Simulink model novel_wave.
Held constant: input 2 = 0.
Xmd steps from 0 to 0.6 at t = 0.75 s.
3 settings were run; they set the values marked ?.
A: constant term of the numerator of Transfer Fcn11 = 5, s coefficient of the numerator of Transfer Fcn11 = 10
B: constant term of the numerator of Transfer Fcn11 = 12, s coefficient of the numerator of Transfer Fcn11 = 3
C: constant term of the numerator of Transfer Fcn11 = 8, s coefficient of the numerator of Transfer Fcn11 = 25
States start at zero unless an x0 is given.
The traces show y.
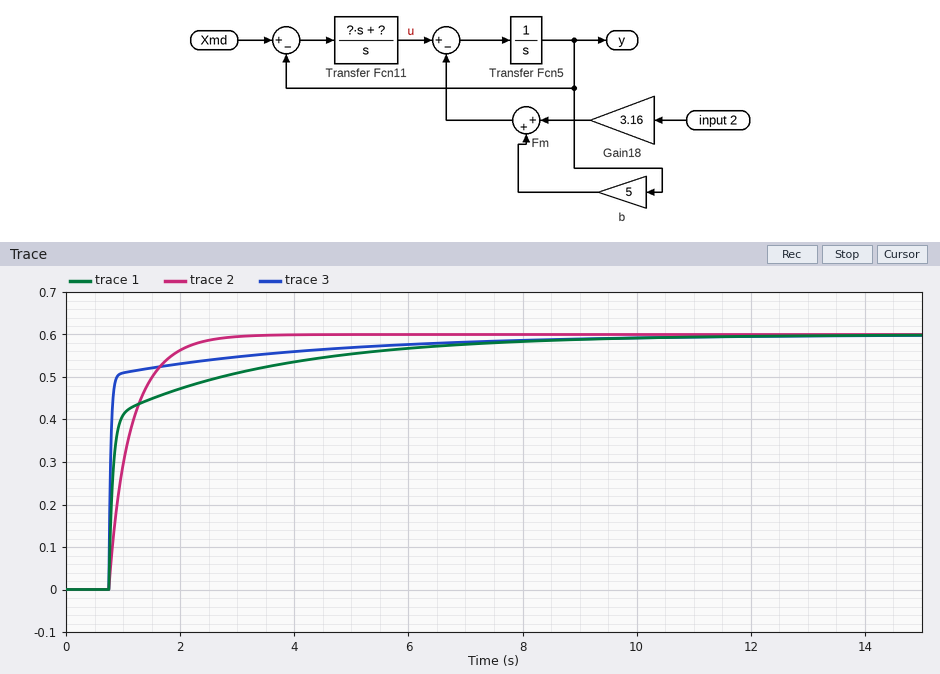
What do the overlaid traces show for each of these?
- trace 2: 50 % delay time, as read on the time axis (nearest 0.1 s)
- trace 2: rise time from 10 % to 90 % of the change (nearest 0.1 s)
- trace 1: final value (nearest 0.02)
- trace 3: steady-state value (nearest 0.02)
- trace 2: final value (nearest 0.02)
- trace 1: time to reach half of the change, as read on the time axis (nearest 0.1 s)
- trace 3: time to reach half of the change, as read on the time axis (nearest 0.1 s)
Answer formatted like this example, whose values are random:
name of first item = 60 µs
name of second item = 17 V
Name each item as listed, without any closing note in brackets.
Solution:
trace 2: 50 % delay time, as read on the time axis = 1.0 s
trace 2: rise time from 10 % to 90 % of the change = 1.0 s
trace 1: final value = 0.60
trace 3: steady-state value = 0.60
trace 2: final value = 0.60
trace 1: time to reach half of the change, as read on the time axis = 0.8 s
trace 3: time to reach half of the change, as read on the time axis = 0.8 s
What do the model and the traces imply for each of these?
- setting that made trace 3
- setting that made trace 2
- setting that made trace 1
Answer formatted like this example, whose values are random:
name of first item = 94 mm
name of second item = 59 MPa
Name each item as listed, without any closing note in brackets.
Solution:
setting that made trace 3 = C
setting that made trace 2 = B
setting that made trace 1 = A
